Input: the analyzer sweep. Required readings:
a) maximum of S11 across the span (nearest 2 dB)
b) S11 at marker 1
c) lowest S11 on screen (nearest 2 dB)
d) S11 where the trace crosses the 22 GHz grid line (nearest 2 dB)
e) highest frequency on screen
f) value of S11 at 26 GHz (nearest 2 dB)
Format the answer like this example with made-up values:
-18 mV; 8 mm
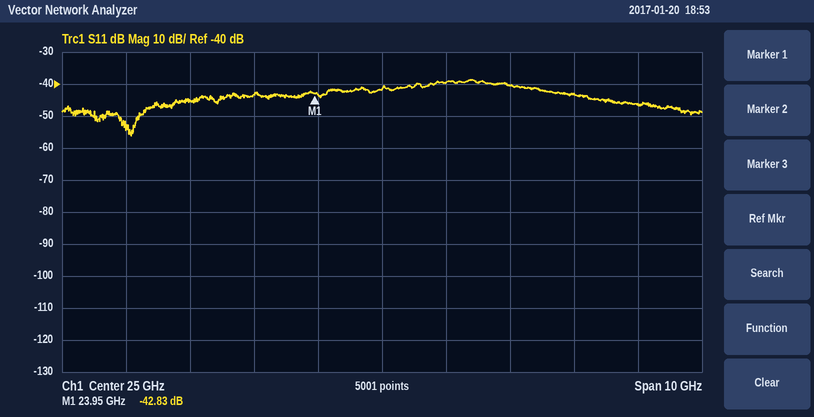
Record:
-38 dB; -42.83 dB; -56 dB; -46 dB; 30 GHz; -40 dB
